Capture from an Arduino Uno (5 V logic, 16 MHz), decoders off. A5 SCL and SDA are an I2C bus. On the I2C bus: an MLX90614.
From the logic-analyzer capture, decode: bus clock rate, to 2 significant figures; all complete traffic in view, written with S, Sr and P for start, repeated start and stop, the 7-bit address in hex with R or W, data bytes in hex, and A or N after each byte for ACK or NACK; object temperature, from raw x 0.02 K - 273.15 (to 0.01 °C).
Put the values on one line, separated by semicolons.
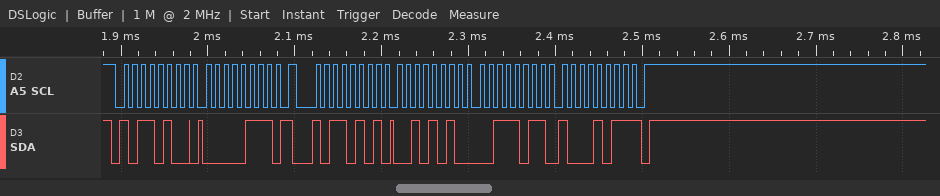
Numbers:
100 kHz; S 5AW A 07 A Sr 5AR A 2A A 3B A 8B N P; 29.77 °C
